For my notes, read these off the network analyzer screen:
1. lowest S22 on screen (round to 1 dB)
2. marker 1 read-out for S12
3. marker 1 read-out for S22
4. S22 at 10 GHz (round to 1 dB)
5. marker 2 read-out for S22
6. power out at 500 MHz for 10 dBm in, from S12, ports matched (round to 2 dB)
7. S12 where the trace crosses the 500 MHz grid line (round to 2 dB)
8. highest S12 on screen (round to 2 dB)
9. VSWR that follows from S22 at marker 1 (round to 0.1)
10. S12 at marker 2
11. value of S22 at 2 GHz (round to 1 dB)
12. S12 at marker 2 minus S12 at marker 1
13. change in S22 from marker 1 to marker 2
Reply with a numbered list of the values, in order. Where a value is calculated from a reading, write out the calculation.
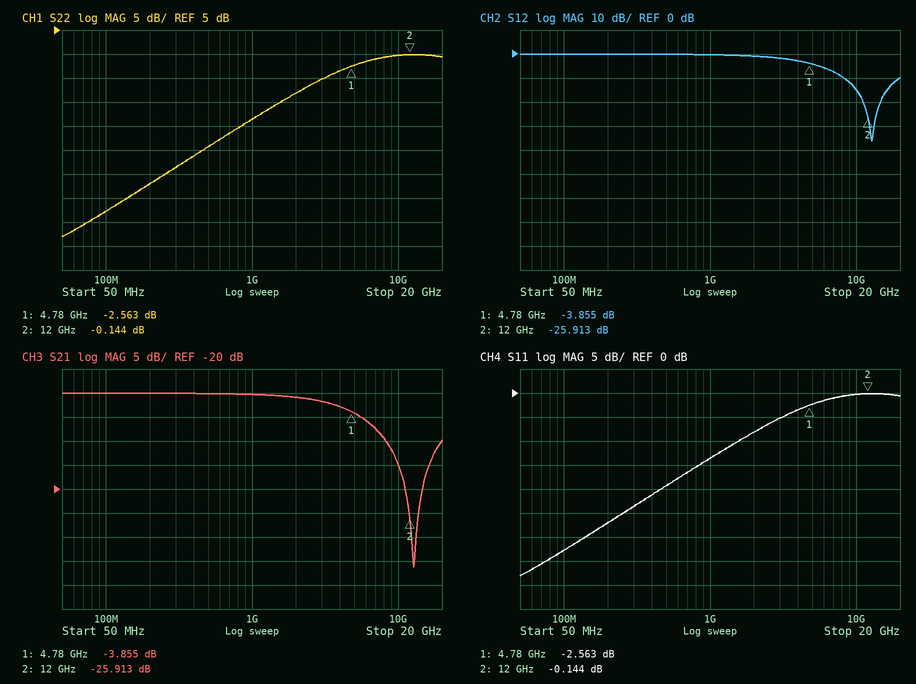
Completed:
1. -38 dB
2. -3.855 dB
3. -2.563 dB
4. 0 dB
5. -0.144 dB
6. 10 dBm + (0 dB) = 10 dBm
7. 0 dB
8. 0 dB
9. (1 + 0.7445)/(1 − 0.7445) ≈ 6.8
10. -25.913 dB
11. -8 dB
12. -25.913 − (-3.855) = -22.058 dB
13. -0.144 − (-2.563) = 2.419 dB
